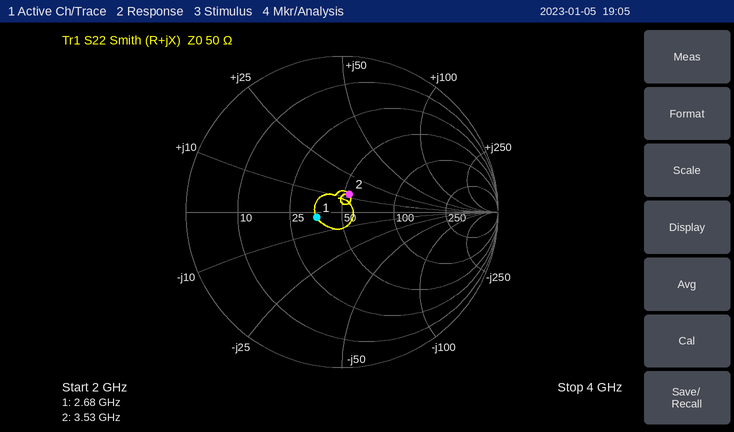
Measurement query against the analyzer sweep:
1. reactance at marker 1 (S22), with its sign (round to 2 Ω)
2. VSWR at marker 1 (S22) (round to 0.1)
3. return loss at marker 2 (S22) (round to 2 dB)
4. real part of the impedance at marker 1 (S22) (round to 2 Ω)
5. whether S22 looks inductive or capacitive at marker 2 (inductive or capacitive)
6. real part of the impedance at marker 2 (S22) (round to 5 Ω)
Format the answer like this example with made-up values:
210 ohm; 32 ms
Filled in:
-2 Ω; 1.4; 18 dB; 36 Ω; inductive; 55 Ω
